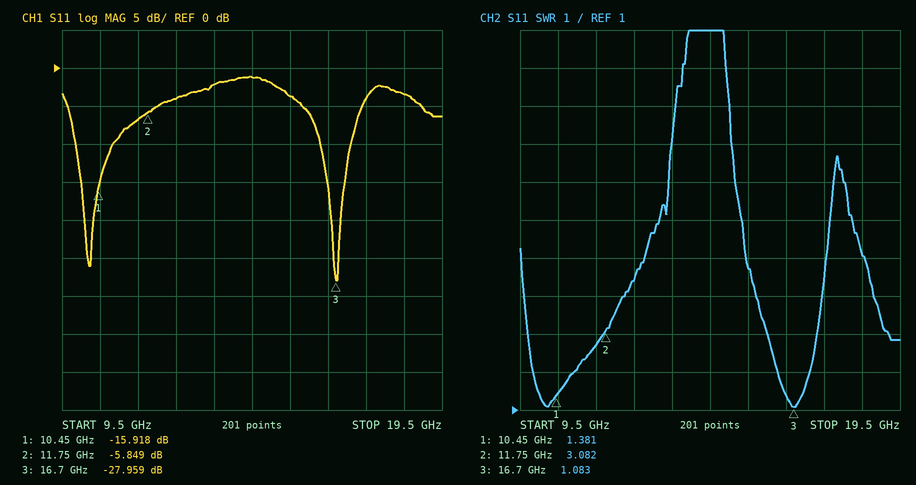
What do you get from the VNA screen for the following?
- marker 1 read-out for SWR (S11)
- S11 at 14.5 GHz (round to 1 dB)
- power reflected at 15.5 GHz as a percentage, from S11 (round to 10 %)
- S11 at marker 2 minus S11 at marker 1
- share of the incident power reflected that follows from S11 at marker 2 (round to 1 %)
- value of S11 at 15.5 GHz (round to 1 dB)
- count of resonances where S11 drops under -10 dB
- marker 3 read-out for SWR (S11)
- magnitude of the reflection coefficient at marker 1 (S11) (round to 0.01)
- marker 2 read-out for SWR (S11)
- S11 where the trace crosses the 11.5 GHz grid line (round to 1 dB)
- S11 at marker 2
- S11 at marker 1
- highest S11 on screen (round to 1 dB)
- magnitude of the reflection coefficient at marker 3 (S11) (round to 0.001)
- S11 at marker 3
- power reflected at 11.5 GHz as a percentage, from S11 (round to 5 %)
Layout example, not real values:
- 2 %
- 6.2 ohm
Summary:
- 1.381
- -1 dB
- 40 %
- 10.069 dB
- 26 %
- -4 dB
- 2
- 1.083
- 0.16
- 3.082
- -7 dB
- -5.849 dB
- -15.918 dB
- -1 dB
- 0.040
- -27.959 dB
- 20 %
